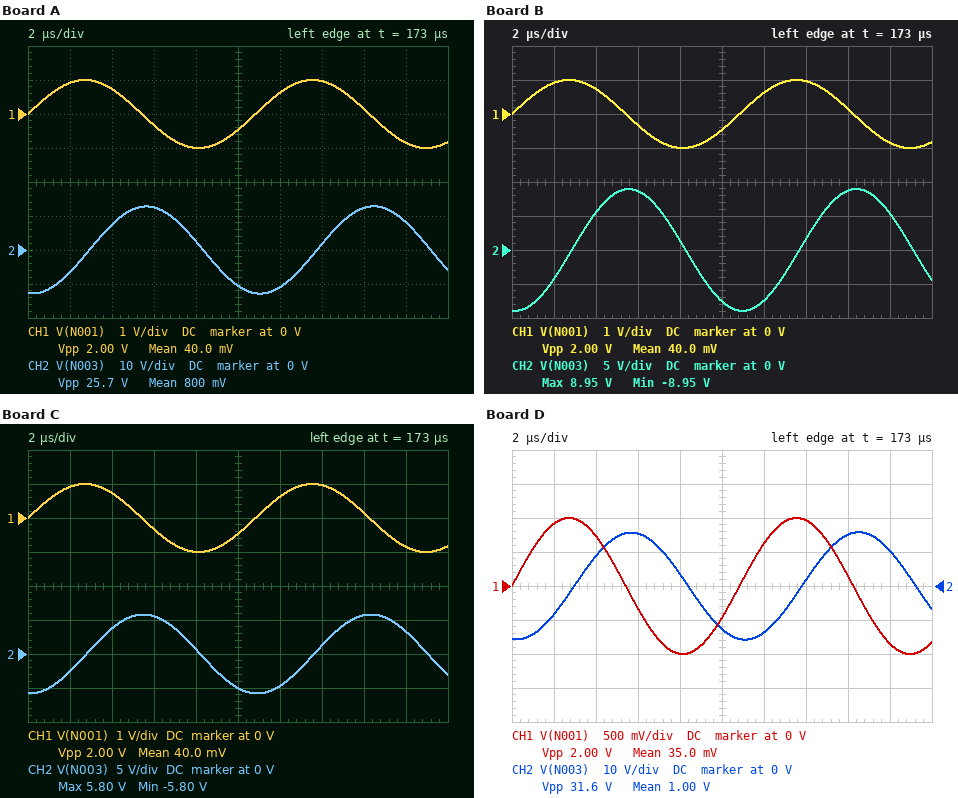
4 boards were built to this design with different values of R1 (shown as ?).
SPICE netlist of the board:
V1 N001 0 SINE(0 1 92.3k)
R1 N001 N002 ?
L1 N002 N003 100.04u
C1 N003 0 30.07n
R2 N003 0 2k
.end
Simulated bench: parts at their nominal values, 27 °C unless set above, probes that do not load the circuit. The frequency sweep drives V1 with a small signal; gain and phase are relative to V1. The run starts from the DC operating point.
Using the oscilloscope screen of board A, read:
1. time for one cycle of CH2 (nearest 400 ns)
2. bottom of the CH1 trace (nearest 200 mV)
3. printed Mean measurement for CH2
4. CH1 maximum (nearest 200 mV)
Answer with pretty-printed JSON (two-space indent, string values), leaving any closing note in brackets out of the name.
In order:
{
  "time for one cycle of CH2": "10.8 µs",
  "bottom of the CH1 trace": "-1.0 V",
  "printed Mean measurement for CH2": "800 mV",
  "CH1 maximum": "1.0 V"
}
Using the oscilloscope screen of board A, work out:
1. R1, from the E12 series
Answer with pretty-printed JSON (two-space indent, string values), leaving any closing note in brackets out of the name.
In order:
{
  "R1, from the E12 series": "2.7 Ω"
}
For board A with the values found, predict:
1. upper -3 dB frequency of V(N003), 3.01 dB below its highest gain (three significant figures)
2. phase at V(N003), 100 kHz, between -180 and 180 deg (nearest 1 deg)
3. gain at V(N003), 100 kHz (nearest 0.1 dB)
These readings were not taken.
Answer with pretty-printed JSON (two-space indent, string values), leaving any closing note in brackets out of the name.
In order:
{
  "upper -3 dB frequency of V(N003), 3.01 dB below its highest gain": "95.1 kHz",
  "phase at V(N003), 100 kHz, between -180 and 180 deg": "-156 deg",
  "gain at V(N003), 100 kHz": "13.8 dB"
}
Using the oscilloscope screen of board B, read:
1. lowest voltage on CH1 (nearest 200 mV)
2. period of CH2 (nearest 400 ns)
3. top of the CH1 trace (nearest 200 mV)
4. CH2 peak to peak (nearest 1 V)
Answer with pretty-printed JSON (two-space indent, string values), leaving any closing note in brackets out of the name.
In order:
{
  "lowest voltage on CH1": "-1.0 V",
  "period of CH2": "10.8 µs",
  "top of the CH1 trace": "1.0 V",
  "CH2 peak to peak": "18 V"
}
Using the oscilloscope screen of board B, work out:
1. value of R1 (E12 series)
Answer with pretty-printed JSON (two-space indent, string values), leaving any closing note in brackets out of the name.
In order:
{
  "value of R1": "4.7 Ω"
}
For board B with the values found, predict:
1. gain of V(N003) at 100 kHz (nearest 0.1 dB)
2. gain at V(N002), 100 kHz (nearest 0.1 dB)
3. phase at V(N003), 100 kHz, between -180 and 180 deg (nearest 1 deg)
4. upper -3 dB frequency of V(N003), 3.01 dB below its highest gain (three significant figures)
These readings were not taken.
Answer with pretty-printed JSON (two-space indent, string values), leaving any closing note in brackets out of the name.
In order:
{
  "gain of V(N003) at 100 kHz": "13.1 dB",
  "gain at V(N002), 100 kHz": "-1.3 dB",
  "phase at V(N003), 100 kHz, between -180 and 180 deg": "-147 deg",
  "upper -3 dB frequency of V(N003), 3.01 dB below its highest gain": "96.5 kHz"
}
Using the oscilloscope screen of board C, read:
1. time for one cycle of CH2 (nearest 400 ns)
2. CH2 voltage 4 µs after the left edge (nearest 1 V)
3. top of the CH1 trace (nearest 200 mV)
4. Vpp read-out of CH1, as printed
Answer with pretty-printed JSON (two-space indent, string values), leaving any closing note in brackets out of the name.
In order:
{
  "time for one cycle of CH2": "10.8 µs",
  "CH2 voltage 4 µs after the left edge": "4 V",
  "top of the CH1 trace": "1.0 V",
  "Vpp read-out of CH1, as printed": "2.00 V"
}
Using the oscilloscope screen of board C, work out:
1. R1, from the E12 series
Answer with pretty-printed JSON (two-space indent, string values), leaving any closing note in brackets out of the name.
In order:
{
  "R1, from the E12 series": "8.2 Ω"
}
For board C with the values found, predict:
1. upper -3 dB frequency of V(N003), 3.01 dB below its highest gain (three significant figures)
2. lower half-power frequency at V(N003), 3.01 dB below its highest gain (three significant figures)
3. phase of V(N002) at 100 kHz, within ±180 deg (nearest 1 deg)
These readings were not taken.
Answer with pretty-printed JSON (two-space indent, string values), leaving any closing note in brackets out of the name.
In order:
{
  "upper -3 dB frequency of V(N003), 3.01 dB below its highest gain": "98.8 kHz",
  "lower half-power frequency at V(N003), 3.01 dB below its highest gain": "83.0 kHz",
  "phase of V(N002) at 100 kHz, within ±180 deg": "36 deg"
}
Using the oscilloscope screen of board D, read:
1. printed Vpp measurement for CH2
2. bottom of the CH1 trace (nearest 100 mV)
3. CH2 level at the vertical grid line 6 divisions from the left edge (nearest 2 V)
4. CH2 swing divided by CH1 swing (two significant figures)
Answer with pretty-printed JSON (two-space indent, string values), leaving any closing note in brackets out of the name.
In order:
{
  "printed Vpp measurement for CH2": "31.6 V",
  "bottom of the CH1 trace": "-1.0 V",
  "CH2 level at the vertical grid line 6 divisions from the left edge": "-14 V",
  "CH2 swing divided by CH1 swing": "16"
}
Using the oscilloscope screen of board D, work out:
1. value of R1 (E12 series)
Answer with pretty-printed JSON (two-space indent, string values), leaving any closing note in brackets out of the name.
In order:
{
  "value of R1": "1.8 Ω"
}
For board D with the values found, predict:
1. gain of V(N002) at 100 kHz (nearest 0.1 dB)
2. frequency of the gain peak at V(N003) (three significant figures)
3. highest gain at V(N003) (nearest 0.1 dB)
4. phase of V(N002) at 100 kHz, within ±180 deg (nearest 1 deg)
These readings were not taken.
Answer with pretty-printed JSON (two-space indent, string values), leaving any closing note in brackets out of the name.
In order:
{
  "gain of V(N002) at 100 kHz": "-0.3 dB",
  "frequency of the gain peak at V(N003)": "91.7 kHz",
  "highest gain at V(N003)": "24.4 dB",
  "phase of V(N002) at 100 kHz, within ±180 deg": "10 deg"
}
